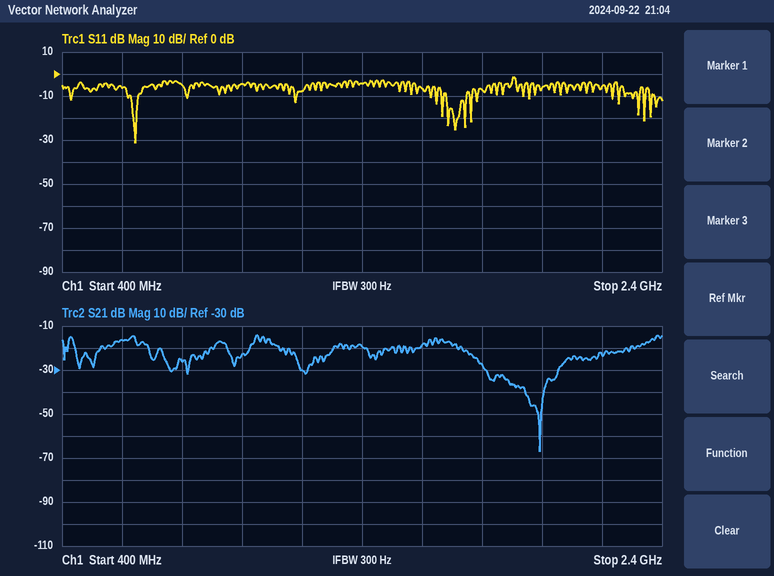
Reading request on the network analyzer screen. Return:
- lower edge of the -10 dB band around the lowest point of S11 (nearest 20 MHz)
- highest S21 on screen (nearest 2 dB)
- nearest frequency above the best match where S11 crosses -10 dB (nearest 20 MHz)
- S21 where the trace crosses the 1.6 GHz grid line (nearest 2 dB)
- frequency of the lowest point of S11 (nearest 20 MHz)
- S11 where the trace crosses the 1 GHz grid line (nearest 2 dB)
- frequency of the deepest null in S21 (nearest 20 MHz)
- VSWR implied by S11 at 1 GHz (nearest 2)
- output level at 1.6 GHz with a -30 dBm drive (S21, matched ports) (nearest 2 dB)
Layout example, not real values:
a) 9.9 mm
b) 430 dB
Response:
a) 620 MHz
b) -14 dB
c) 660 MHz
d) -18 dB
e) 640 MHz
f) -4 dB
g) 2.00 GHz
h) 4
i) -48 dBm
